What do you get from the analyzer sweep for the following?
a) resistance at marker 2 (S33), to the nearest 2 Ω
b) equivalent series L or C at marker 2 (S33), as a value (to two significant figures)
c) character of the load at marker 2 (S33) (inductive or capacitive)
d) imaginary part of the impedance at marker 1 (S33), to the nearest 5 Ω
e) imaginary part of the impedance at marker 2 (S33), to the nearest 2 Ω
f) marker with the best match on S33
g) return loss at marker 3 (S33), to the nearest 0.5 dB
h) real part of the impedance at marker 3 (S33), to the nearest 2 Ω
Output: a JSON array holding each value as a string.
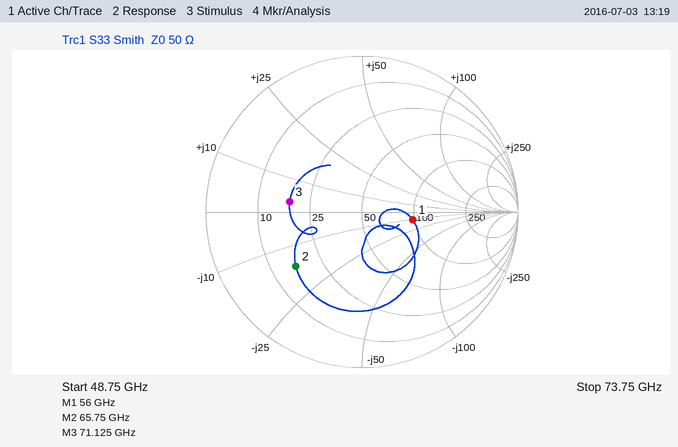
["16 Ω", "150 fF", "capacitive", "-10 Ω", "-16 Ω", "marker 1", "6.5 dB", "18 Ω"]
